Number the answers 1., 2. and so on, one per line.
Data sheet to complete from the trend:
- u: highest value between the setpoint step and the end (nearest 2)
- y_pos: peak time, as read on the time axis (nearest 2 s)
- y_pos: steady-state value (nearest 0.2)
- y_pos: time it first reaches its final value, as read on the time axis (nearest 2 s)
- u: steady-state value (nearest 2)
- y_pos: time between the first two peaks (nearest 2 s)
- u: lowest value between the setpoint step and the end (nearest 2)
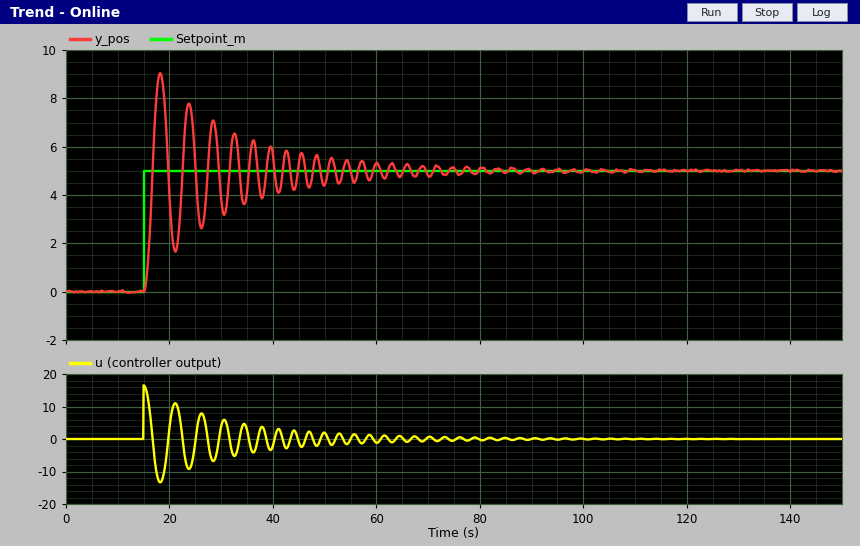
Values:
1. 16
2. 18 s
3. 5.0
4. 16 s
5. 0
6. 6 s
7. -14
